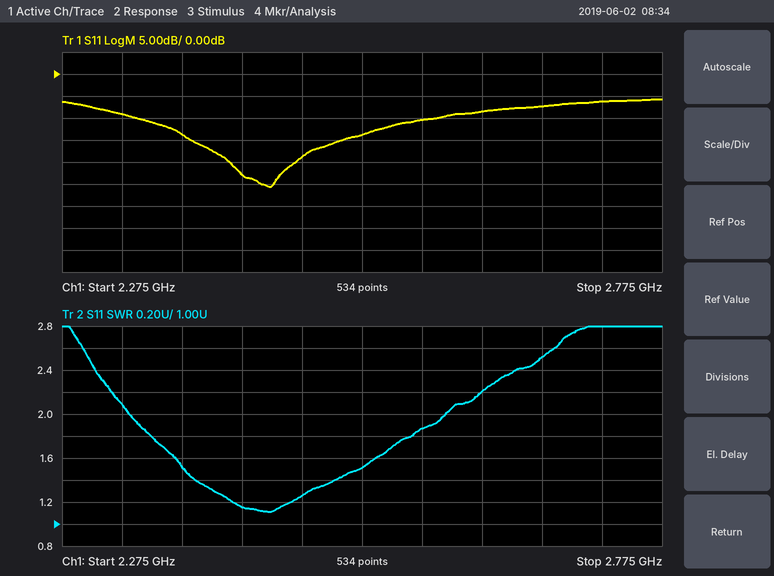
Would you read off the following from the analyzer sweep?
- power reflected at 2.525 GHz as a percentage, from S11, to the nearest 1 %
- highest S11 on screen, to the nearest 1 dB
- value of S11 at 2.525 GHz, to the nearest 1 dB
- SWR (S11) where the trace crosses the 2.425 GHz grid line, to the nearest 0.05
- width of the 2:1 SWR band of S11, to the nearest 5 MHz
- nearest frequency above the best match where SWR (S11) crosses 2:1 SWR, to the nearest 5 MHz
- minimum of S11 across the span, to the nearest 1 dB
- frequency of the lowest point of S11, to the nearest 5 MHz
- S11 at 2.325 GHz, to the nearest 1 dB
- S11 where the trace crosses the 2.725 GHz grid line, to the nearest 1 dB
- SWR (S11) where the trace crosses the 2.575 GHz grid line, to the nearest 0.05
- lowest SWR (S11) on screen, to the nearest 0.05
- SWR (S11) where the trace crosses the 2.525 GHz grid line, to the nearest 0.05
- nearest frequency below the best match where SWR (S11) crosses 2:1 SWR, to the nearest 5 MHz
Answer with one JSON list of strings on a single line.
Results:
["4 %", "-6 dB", "-14 dB", "1.15", "265 MHz", "2.595 GHz", "-26 dB", "2.450 GHz", "-9 dB", "-6 dB", "1.85", "1.10", "1.50", "2.330 GHz"]
